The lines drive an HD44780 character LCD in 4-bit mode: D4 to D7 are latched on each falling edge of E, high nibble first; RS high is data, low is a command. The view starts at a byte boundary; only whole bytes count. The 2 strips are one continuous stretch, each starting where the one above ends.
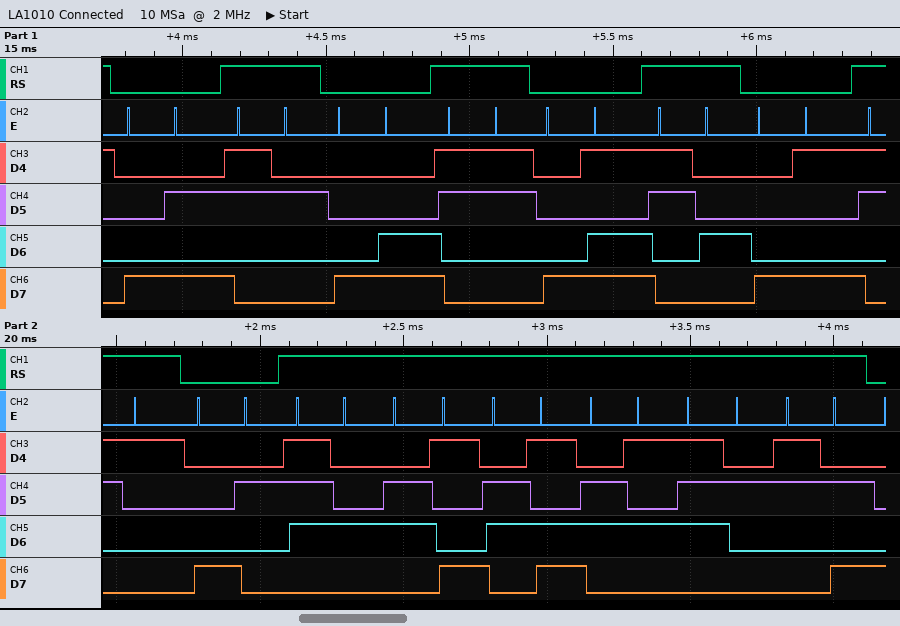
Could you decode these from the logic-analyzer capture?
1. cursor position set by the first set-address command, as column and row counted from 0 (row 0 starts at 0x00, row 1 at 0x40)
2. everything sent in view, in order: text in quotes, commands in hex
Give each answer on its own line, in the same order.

column 10, row 0
0x8A "2" 0x8C "3" 0x8D "4" 0x89 "1" 0x82 "timer:"
